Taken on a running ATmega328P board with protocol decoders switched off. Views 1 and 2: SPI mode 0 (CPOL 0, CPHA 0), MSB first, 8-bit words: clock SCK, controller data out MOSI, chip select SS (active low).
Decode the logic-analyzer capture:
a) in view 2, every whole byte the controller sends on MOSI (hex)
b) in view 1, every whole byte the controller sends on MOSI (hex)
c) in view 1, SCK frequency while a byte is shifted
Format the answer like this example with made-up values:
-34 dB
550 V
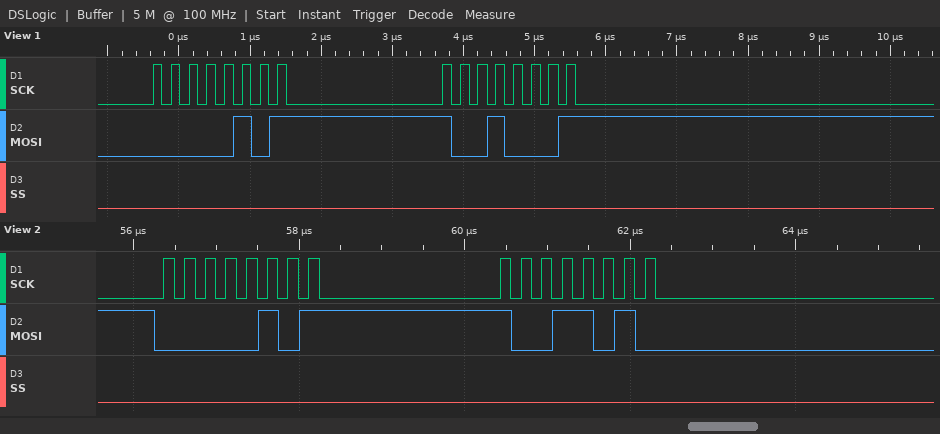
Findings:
05 9A
05 91
4 MHz
